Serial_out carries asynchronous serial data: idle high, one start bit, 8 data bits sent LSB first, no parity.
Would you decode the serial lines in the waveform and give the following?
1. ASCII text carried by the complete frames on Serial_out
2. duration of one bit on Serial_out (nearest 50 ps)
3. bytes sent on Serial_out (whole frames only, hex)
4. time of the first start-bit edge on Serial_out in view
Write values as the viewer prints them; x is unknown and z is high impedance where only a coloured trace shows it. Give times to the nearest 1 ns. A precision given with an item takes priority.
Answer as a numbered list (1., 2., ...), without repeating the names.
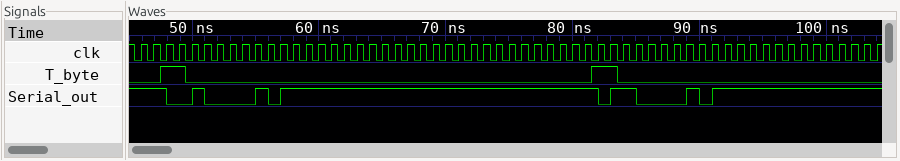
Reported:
1. "BC"
2. 1000 ps
3. 42, 43
4. 48 ns
